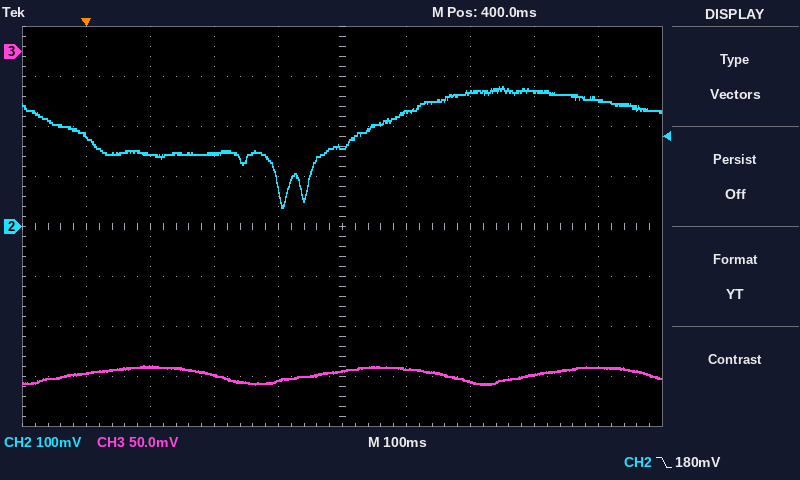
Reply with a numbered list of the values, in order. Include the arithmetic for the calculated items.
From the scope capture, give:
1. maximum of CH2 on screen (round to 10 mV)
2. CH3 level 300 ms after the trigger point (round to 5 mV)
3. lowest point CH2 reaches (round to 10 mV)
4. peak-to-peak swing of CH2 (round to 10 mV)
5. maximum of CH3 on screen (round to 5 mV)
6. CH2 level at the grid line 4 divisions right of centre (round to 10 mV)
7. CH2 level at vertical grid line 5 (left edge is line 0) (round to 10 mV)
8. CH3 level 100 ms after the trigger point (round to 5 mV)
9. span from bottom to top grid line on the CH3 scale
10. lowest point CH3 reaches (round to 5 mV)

1. 280 mV
2. -330 mV
3. 40 mV
4. 280 mV − (40 mV) = 240 mV
5. -315 mV
6. 250 mV
7. 160 mV
8. -315 mV
9. 400 mV
10. -335 mV
